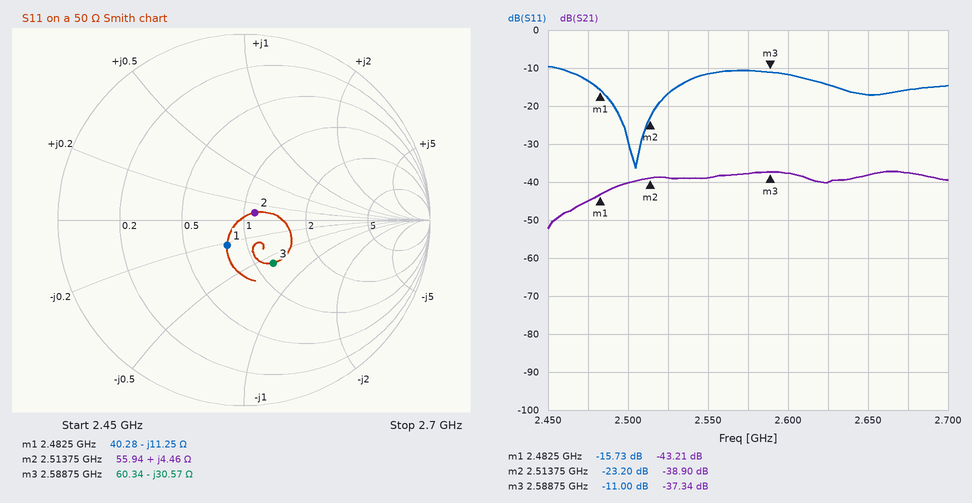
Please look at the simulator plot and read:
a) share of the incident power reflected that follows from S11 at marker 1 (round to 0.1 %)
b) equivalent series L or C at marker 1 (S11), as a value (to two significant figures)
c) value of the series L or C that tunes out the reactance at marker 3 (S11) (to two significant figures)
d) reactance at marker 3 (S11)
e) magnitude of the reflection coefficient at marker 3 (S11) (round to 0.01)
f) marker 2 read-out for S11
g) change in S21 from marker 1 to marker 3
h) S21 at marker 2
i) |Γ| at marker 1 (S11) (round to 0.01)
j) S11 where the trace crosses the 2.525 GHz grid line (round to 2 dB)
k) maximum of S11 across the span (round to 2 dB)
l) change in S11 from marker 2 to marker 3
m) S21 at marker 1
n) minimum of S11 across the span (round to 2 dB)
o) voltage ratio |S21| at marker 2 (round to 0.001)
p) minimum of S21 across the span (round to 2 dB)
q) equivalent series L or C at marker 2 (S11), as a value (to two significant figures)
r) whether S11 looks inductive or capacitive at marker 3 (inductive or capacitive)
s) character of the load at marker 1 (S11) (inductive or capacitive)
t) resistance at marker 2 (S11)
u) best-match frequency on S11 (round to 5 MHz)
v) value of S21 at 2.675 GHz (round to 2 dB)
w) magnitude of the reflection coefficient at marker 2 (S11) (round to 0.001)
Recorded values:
2.7 %
5.7 pF
1.9 nH
-30.57 Ω
0.28
-23.20 dB
5.87 dB
-38.90 dB
0.16
-16 dB
-10 dB
12.20 dB
-43.21 dB
-36 dB
0.011
-52 dB
280 pH
capacitive
capacitive
55.94 Ω
2.505 GHz
-38 dB
0.069
